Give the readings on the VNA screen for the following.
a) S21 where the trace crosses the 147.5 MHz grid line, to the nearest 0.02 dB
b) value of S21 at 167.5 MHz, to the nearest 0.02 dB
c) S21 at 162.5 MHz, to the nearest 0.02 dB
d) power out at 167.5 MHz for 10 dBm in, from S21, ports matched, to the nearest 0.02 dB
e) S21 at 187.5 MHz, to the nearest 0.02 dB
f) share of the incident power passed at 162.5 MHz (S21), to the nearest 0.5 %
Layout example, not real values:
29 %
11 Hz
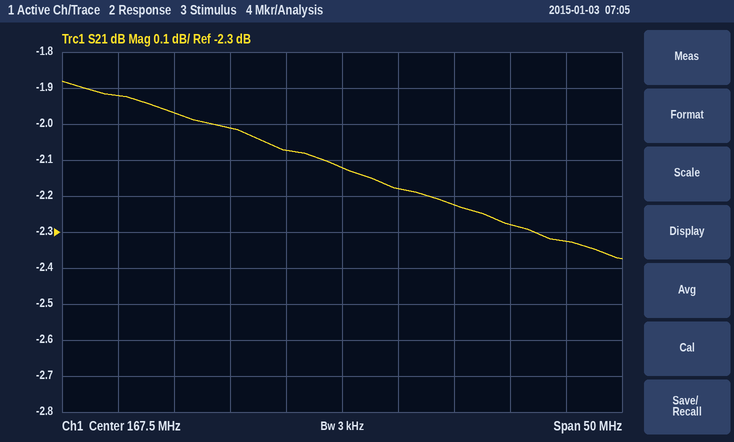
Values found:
-1.92 dB
-2.12 dB
-2.08 dB
7.88 dBm
-2.32 dB
62.0 %
